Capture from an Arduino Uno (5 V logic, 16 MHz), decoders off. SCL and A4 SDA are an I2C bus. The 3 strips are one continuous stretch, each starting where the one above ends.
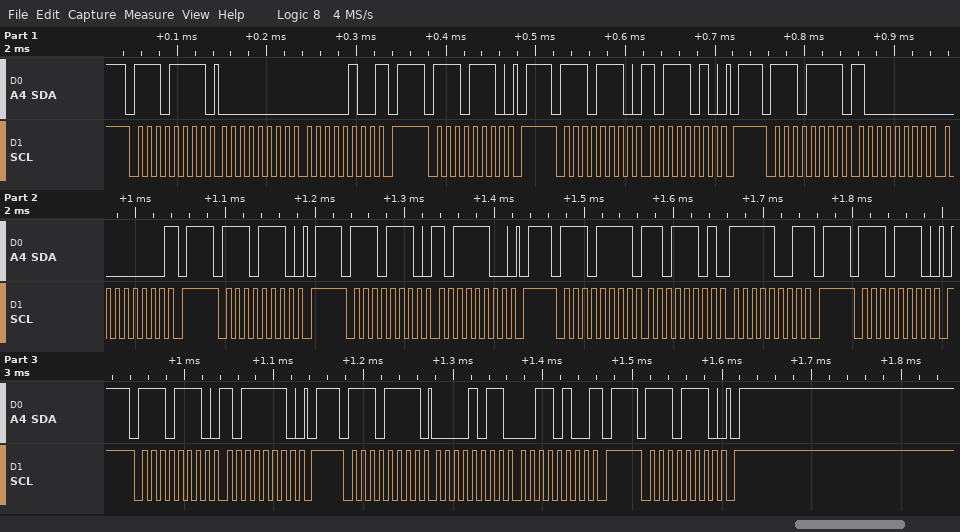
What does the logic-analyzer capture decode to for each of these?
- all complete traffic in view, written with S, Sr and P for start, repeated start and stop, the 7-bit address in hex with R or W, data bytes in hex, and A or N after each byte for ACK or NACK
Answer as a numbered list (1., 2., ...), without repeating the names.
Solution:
1. S 77R A 00 A 04 N P S 77W A P S 77W A BA A P S 77R A 80 A 00 N P S 77W A P S 77W A BC A P S 77R A DD A F9 N P S 77W A P S 77W A BE A P S 77R A 0B A 34 N P S 77W A P
